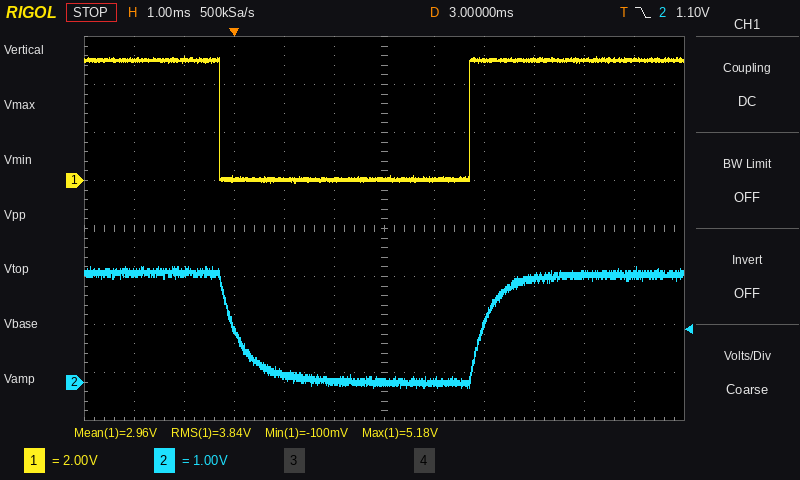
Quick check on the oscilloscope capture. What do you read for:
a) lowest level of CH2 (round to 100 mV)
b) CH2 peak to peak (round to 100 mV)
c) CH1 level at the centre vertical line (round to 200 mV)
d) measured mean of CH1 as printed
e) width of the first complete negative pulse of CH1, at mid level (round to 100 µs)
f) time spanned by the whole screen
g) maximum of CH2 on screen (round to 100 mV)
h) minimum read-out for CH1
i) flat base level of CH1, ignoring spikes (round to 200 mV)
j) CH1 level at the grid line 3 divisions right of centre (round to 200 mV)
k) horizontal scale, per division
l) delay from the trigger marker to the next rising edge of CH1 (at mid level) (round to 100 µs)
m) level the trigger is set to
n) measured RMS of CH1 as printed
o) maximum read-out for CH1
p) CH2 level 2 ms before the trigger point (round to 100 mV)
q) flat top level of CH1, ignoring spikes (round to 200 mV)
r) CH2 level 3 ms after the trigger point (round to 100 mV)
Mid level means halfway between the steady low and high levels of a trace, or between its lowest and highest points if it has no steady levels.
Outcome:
-100 mV
2.5 V
0.0 V
2.96 V
5.0 ms
12 ms
2.4 V
-100 mV
0.0 V
5.0 V
1 ms
4.7 ms
1.10 V
3.84 V
5.18 V
2.3 V
5.0 V
0.0 V
